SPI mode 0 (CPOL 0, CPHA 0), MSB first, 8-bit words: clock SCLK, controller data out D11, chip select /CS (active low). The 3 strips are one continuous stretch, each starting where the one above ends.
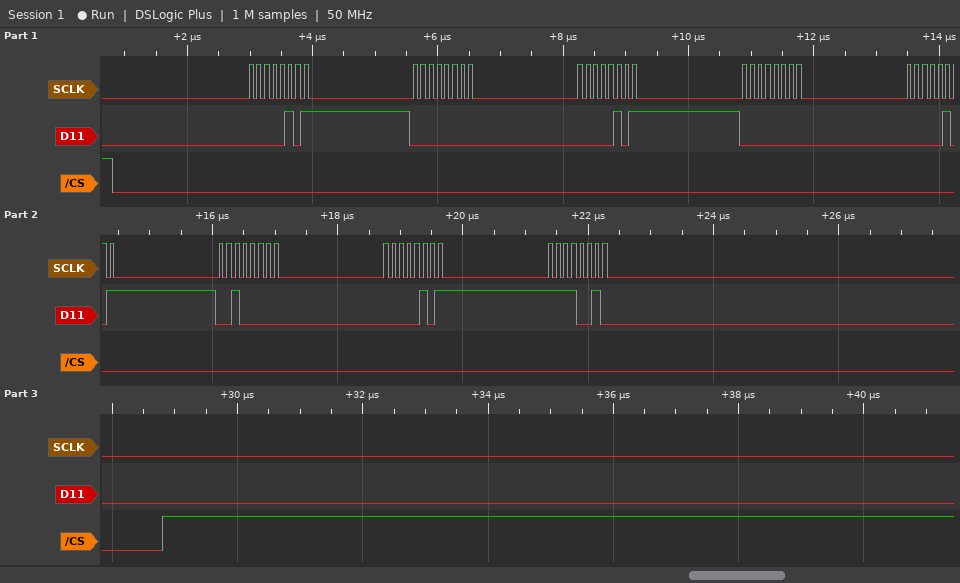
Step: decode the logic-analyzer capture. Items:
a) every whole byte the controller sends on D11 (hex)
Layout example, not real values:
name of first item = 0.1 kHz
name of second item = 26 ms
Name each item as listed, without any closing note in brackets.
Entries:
every whole byte the controller sends on D11 = 0x05 0x00 0x05 0x00 0x05 0x20 0x05 0xF2
